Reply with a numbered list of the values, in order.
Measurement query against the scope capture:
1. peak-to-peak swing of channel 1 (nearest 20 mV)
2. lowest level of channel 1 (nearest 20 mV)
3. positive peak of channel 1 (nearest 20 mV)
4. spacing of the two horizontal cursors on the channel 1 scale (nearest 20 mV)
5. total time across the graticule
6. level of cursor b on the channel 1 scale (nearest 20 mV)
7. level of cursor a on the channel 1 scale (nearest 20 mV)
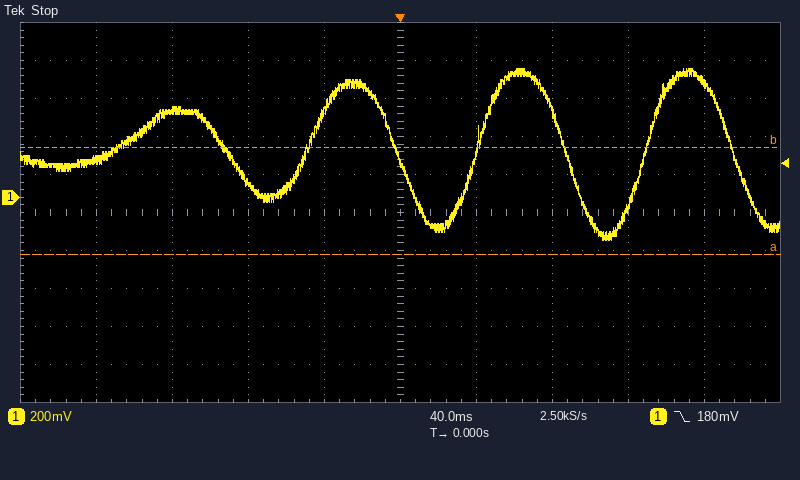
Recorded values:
1. 900 mV
2. -220 mV
3. 680 mV
4. 560 mV
5. 400 ms
6. 260 mV
7. -300 mV
